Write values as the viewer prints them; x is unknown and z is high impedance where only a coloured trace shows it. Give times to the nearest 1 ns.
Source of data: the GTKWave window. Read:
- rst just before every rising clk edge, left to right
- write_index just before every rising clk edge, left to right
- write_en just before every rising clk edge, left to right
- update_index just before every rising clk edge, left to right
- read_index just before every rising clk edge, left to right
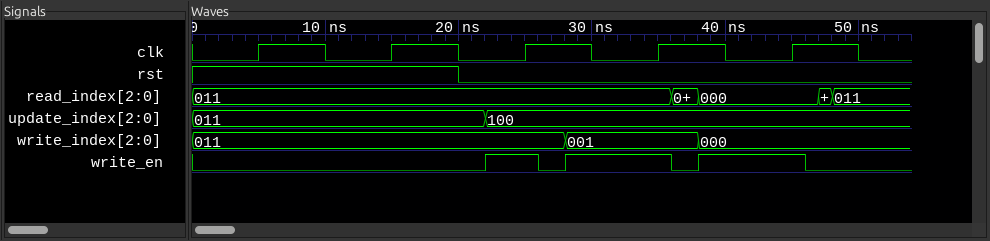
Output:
1 1 0 0 0
011, 011, 011, 001, 000
0 0 1 1 1
011, 011, 100, 100, 100
011, 011, 011, 011, 000
